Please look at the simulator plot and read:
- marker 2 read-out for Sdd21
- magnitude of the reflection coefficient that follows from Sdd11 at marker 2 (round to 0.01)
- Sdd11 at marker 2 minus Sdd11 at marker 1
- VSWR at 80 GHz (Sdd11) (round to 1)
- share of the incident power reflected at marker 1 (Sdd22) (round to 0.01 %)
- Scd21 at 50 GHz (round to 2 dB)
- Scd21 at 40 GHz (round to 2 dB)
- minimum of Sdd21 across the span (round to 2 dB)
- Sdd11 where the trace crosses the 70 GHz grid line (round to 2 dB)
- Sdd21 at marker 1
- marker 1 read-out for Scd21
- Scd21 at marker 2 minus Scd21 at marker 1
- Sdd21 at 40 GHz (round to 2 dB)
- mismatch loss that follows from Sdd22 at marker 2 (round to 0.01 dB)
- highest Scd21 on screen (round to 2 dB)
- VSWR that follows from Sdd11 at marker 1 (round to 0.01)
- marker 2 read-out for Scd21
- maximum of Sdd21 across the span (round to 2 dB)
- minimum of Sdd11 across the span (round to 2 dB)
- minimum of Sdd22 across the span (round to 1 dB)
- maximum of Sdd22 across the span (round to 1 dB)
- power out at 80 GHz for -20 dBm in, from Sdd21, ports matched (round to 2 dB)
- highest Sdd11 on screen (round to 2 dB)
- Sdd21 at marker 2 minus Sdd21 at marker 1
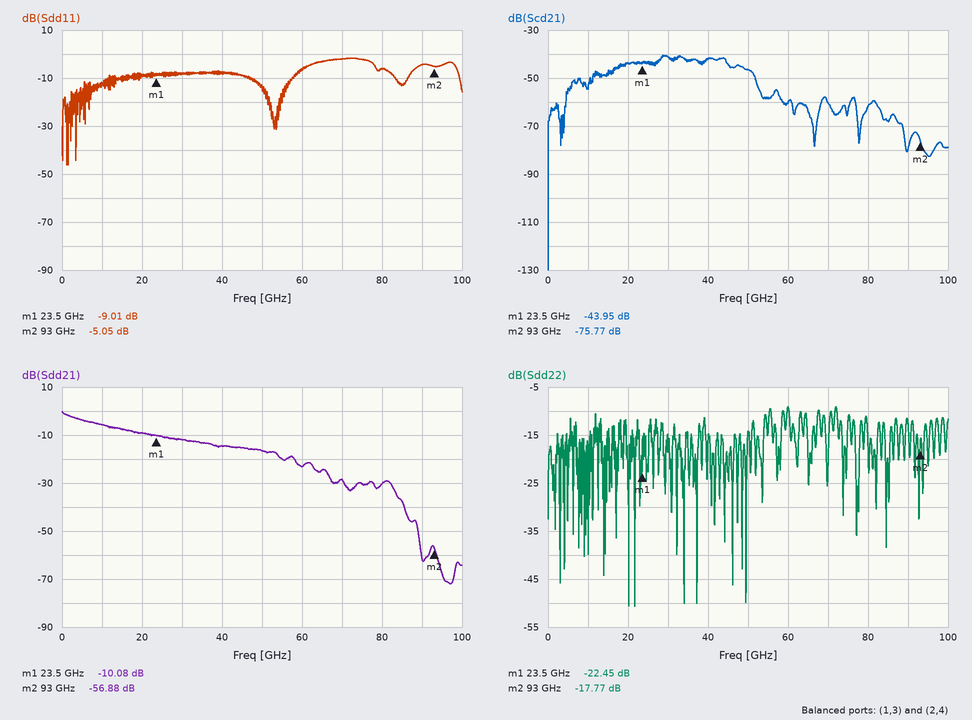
-56.88 dB
0.56
3.96 dB
3
0.57 %
-46 dB
-42 dB
-72 dB
-2 dB
-10.08 dB
-43.95 dB
-31.82 dB
-14 dB
0.07 dB
-40 dB
2.10
-75.77 dB
0 dB
-46 dB
-51 dB
-9 dB
-50 dBm
-2 dB
-46.80 dB
